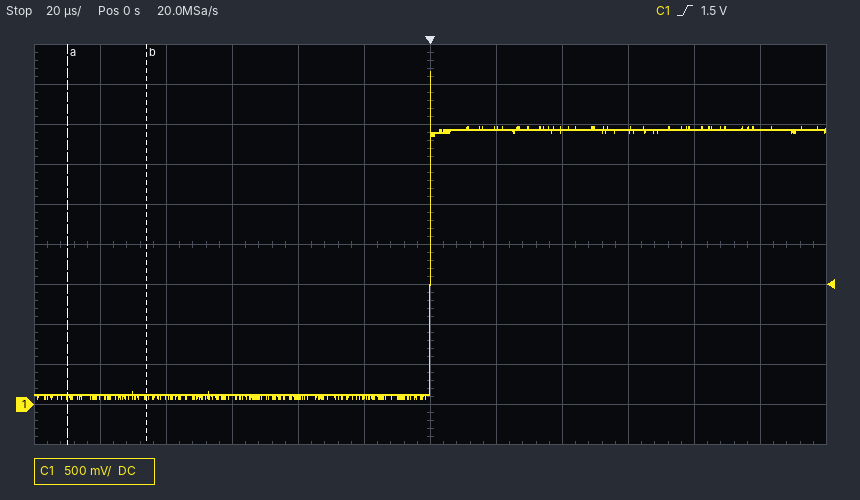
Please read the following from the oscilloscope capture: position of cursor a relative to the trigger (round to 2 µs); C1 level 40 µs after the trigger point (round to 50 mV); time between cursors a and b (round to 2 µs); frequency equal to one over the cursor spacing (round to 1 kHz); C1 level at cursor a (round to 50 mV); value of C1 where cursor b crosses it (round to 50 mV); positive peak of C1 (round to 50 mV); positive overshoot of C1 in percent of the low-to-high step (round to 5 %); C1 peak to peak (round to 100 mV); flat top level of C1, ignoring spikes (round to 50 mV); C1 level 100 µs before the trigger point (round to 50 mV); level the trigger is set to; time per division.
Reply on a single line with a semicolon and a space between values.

-110 µs; 3.45 V; 24 µs; 42 kHz; 100 mV; 100 mV; 4.15 V; 20 %; 4.10 V; 3.45 V; 100 mV; 1.5 V; 20 µs
